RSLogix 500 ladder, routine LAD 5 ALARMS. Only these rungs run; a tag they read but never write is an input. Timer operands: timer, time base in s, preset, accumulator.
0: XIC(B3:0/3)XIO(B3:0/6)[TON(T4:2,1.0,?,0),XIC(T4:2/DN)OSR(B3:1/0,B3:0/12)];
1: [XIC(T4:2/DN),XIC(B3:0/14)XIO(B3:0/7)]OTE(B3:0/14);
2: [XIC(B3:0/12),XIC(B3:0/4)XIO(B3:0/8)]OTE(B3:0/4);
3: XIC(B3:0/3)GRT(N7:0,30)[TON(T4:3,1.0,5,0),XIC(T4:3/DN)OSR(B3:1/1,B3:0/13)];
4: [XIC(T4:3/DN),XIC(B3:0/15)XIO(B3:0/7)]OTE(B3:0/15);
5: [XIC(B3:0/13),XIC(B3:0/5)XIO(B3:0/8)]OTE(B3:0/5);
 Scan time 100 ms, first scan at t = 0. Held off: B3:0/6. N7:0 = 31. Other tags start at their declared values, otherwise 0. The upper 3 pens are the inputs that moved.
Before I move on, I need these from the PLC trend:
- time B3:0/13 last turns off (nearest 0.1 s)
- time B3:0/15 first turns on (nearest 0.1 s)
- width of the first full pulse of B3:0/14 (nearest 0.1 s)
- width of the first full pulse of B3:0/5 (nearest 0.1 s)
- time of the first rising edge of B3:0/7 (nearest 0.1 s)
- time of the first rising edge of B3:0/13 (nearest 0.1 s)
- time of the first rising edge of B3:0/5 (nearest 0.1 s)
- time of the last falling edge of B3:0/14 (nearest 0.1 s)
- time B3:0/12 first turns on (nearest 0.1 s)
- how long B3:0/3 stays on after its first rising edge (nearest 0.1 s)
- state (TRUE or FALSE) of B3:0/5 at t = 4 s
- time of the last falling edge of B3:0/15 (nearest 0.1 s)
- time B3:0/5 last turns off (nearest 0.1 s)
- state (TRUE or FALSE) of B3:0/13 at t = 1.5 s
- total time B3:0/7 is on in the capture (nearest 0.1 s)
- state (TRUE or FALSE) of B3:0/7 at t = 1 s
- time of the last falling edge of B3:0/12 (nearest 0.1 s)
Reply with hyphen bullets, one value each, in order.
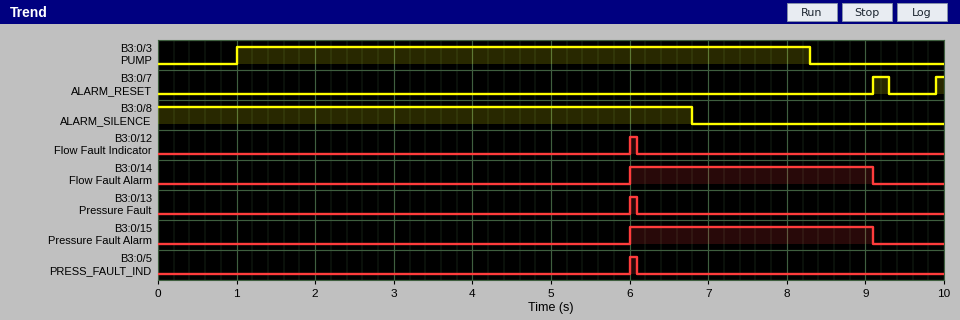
- 6.1 s
- 6.0 s
- 3.1 s
- 0.1 s
- 9.1 s
- 6.0 s
- 6.0 s
- 9.1 s
- 6.0 s
- 7.3 s
- FALSE
- 9.1 s
- 6.1 s
- FALSE
- 0.3 s
- FALSE
- 6.1 s
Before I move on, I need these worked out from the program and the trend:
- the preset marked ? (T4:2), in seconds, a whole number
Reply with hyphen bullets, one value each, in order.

- 5 s
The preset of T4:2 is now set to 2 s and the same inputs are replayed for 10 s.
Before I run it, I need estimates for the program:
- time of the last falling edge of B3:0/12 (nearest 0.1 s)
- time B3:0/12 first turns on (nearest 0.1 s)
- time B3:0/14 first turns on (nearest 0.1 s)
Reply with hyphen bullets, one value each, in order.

- 3.1 s
- 3.0 s
- 3.0 s
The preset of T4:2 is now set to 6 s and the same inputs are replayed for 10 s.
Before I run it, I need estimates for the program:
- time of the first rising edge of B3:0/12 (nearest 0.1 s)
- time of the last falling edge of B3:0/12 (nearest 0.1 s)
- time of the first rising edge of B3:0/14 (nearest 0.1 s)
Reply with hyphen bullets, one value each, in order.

- 7.0 s
- 7.1 s
- 7.0 s
